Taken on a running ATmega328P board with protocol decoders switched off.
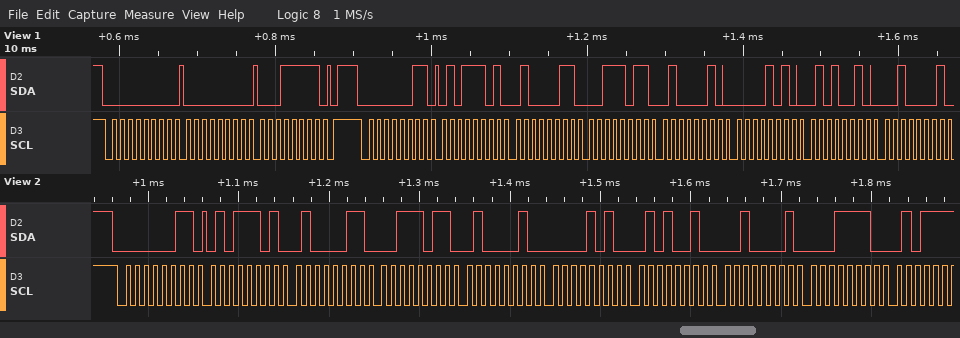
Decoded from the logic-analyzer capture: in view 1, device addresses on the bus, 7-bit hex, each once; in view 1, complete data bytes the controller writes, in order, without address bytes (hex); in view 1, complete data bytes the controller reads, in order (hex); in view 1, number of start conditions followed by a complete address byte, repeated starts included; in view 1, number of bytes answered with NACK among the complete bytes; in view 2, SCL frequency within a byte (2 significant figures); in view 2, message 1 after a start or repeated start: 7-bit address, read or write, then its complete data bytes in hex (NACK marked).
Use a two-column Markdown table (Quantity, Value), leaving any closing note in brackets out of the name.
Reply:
| Quantity | Value |
|---|---|
| in view 1, device addresses on the bus, 7-bit hex, each once | 0x00 0x01 |
| in view 1, complete data bytes the controller writes, in order, without address bytes | 00 1F |
| in view 1, complete data bytes the controller reads, in order | 5D 43 3B 42 0A 52 21 |
| in view 1, number of start conditions followed by a complete address byte, repeated starts included | 2 |
| in view 1, number of bytes answered with NACK among the complete bytes | 0 |
| in view 2, SCL frequency within a byte | 100 kHz |
| in view 2, message 1 after a start or repeated start: 7-bit address, read or write, then its complete data bytes in hex | 0x01 read: 5D 43 3B 42 0A 52 21 1E |
